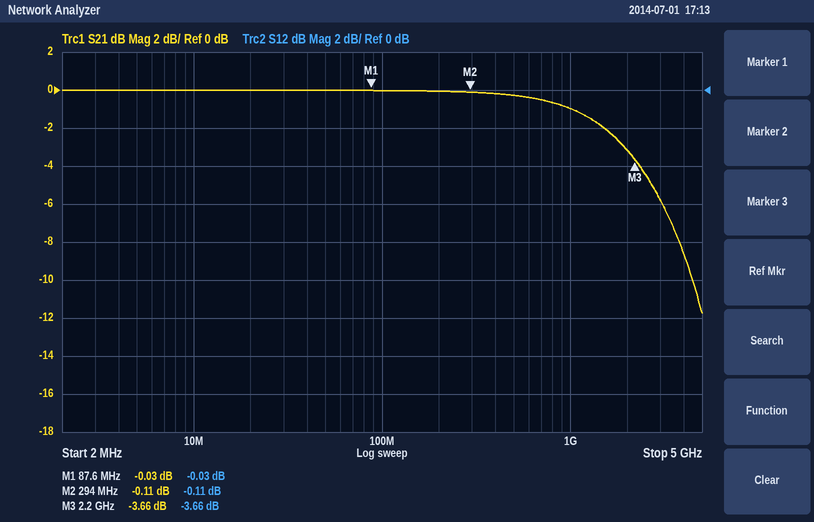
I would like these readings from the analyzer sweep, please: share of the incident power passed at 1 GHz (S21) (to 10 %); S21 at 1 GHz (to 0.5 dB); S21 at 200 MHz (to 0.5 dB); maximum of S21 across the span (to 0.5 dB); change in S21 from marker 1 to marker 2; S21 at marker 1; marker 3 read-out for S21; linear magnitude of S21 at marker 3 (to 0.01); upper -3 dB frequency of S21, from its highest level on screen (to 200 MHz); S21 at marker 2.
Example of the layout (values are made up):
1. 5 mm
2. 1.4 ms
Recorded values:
1. 80 %
2. -1.0 dB
3. 0.0 dB
4. 0.0 dB
5. -0.08 dB
6. -0.03 dB
7. -3.66 dB
8. 0.66
9. 2.0 GHz
10. -0.11 dB
